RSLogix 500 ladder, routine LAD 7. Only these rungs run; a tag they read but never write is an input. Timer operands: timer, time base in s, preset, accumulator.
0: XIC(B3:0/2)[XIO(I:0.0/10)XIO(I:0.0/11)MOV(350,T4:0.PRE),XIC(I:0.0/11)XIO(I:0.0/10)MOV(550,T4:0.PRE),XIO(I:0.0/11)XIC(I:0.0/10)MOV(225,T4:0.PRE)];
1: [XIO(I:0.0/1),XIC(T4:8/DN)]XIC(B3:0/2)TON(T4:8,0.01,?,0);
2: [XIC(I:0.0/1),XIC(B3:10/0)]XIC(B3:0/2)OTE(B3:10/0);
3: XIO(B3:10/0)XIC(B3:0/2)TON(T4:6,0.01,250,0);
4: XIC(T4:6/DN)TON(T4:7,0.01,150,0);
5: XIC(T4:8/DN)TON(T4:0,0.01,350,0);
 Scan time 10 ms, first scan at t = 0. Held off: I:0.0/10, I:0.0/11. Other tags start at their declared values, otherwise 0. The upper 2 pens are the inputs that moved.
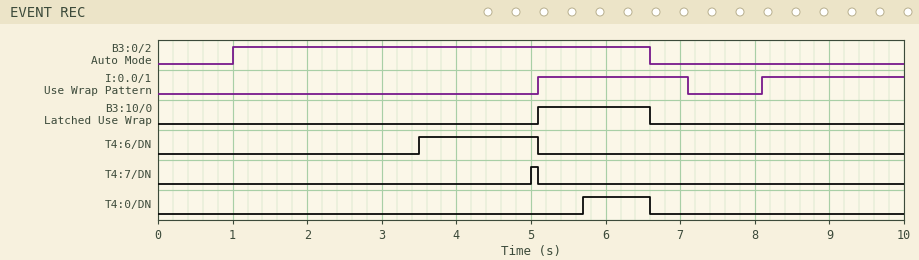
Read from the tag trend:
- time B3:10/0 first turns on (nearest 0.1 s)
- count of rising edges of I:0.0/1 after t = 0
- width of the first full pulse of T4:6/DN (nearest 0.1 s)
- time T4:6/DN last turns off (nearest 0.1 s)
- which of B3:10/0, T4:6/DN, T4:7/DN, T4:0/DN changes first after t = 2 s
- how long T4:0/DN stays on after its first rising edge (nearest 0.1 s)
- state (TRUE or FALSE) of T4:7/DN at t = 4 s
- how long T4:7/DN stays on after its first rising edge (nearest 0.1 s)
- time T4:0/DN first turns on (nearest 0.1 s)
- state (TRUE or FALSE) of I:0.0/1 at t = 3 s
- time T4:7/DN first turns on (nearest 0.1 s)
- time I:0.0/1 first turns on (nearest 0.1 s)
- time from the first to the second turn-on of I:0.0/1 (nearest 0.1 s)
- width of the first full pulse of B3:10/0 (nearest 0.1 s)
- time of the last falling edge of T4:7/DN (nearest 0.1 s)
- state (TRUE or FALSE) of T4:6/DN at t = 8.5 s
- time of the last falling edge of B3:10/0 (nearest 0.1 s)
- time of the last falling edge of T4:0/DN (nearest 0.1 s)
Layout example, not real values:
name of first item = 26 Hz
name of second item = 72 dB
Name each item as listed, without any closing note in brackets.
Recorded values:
time B3:10/0 first turns on = 5.1 s
count of rising edges of I:0.0/1 after t = 0 = 2
width of the first full pulse of T4:6/DN = 1.6 s
time T4:6/DN last turns off = 5.1 s
which of B3:10/0, T4:6/DN, T4:7/DN, T4:0/DN changes first after t = 2 s = T4:6/DN
how long T4:0/DN stays on after its first rising edge = 0.9 s
state (TRUE or FALSE) of T4:7/DN at t = 4 s = FALSE
how long T4:7/DN stays on after its first rising edge = 0.1 s
time T4:0/DN first turns on = 5.7 s
state (TRUE or FALSE) of I:0.0/1 at t = 3 s = FALSE
time T4:7/DN first turns on = 5.0 s
time I:0.0/1 first turns on = 5.1 s
time from the first to the second turn-on of I:0.0/1 = 3.0 s
width of the first full pulse of B3:10/0 = 1.5 s
time of the last falling edge of T4:7/DN = 5.1 s
state (TRUE or FALSE) of T4:6/DN at t = 8.5 s = FALSE
time of the last falling edge of B3:10/0 = 6.6 s
time of the last falling edge of T4:0/DN = 6.6 s
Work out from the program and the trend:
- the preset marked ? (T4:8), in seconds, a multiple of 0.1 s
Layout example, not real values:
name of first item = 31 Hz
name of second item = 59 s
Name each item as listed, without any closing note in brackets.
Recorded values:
the preset marked ? (T4:8), in seconds, a multiple of 0.1 s = 1.2 s
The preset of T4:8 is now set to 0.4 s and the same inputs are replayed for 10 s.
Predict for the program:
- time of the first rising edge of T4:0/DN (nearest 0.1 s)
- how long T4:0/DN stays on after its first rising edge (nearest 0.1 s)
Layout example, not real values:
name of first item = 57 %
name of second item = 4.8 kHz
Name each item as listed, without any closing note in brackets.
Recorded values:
time of the first rising edge of T4:0/DN = 4.9 s
how long T4:0/DN stays on after its first rising edge = 1.7 s
